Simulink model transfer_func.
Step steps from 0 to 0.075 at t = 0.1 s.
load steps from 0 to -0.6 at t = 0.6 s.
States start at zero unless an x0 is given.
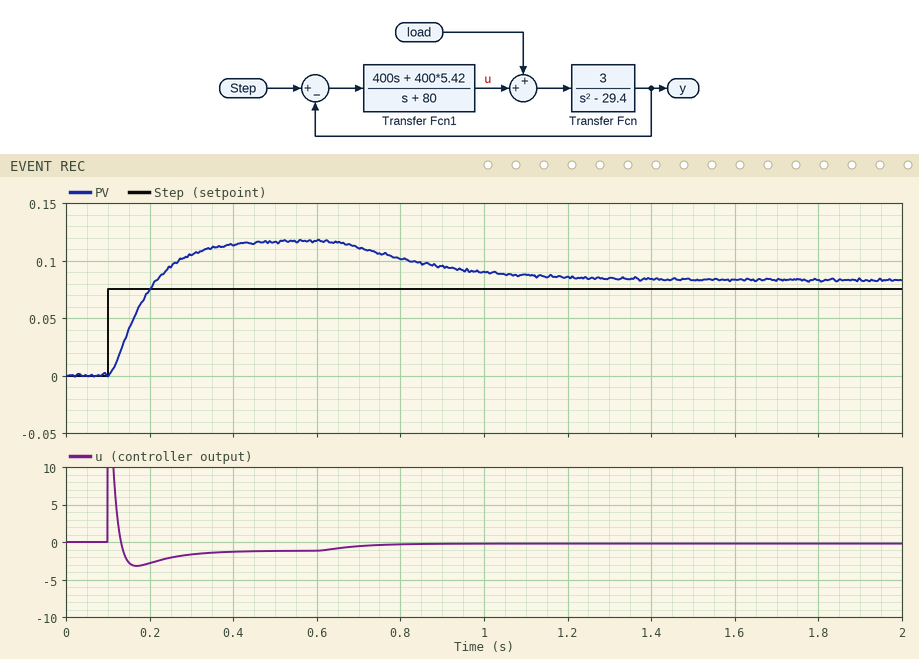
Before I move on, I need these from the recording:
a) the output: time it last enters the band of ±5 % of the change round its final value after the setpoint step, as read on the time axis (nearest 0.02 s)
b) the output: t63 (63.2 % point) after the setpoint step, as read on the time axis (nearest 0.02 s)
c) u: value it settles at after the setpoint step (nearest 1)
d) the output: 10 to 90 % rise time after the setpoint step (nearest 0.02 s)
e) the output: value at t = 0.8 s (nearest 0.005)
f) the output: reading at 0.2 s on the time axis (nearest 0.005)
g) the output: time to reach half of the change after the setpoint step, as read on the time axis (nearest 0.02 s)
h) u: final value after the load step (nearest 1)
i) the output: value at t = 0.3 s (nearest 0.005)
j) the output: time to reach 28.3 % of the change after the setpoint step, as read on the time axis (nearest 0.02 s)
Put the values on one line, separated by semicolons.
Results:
0.36 s; 0.20 s; -1; 0.18 s; 0.100; 0.075; 0.18 s; 0; 0.105; 0.14 s
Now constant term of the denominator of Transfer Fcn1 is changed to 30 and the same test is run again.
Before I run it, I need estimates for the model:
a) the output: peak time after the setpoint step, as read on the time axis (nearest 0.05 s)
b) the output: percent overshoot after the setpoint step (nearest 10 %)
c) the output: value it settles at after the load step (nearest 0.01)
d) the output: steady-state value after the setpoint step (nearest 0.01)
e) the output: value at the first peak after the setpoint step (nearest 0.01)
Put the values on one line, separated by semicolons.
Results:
0.20 s; 30 %; 0.08; 0.09; 0.11
